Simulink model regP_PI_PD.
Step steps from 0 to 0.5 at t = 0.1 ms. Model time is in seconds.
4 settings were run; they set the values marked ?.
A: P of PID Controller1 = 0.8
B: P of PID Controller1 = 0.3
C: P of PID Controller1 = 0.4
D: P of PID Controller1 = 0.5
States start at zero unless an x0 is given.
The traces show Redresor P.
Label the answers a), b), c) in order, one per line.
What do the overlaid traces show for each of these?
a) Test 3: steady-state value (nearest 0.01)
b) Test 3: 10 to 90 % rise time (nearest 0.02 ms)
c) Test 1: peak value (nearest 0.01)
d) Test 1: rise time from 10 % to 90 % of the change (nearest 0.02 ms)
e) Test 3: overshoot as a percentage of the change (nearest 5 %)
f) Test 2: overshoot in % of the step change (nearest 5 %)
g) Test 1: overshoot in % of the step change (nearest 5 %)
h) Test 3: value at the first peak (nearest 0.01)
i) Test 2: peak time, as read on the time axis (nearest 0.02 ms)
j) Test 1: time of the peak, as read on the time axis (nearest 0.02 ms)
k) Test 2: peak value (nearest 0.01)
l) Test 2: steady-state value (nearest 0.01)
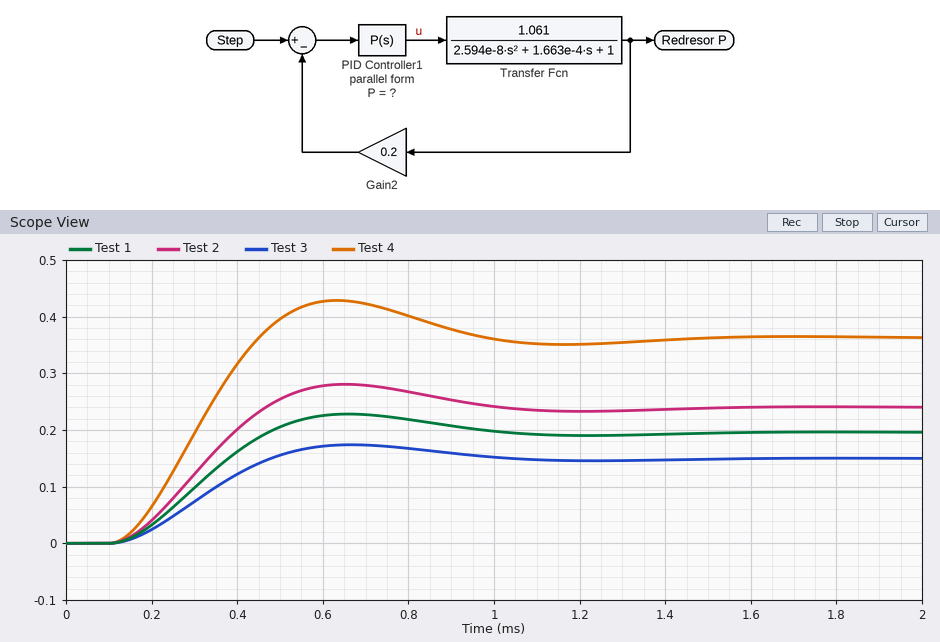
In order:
a) 0.15
b) 0.26 ms
c) 0.23
d) 0.26 ms
e) 15 %
f) 15 %
g) 15 %
h) 0.17
i) 0.66 ms
j) 0.66 ms
k) 0.28
l) 0.24
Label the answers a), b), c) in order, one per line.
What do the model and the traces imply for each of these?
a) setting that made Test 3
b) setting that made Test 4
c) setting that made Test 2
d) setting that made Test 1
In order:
a) B
b) A
c) D
d) C
